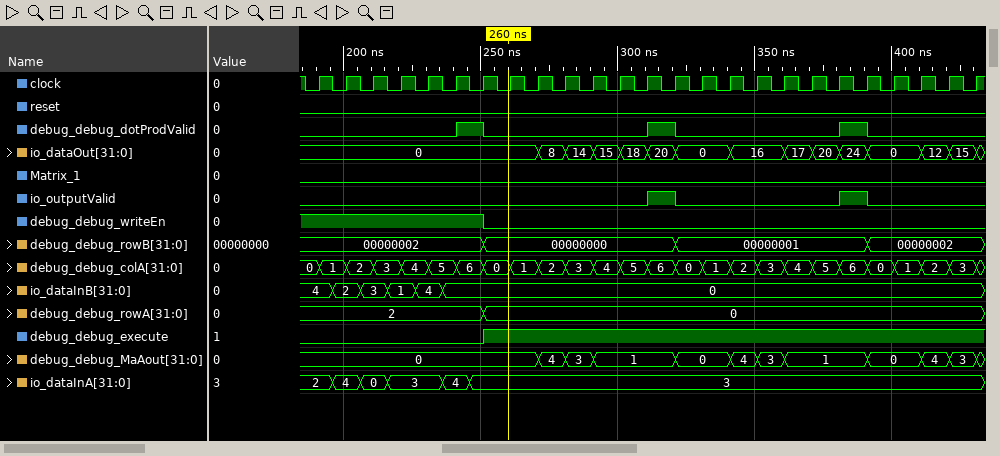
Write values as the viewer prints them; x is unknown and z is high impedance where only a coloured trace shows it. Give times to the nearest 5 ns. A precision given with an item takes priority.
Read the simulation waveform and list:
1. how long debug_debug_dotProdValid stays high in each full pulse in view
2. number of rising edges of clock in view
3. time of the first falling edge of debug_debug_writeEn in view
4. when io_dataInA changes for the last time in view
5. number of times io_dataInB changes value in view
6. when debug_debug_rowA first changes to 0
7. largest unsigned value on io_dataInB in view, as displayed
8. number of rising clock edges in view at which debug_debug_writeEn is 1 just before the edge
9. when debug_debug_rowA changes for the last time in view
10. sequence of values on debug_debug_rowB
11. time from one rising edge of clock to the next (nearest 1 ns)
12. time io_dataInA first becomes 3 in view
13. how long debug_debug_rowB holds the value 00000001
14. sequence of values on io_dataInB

10 ns, 10 ns, 10 ns
25
250 ns
245 ns
5
250 ns
4
7
250 ns
00000002, 00000000, 00000001, 00000002
10 ns
215 ns
70 ns
4, 2, 3, 1, 4, 0
